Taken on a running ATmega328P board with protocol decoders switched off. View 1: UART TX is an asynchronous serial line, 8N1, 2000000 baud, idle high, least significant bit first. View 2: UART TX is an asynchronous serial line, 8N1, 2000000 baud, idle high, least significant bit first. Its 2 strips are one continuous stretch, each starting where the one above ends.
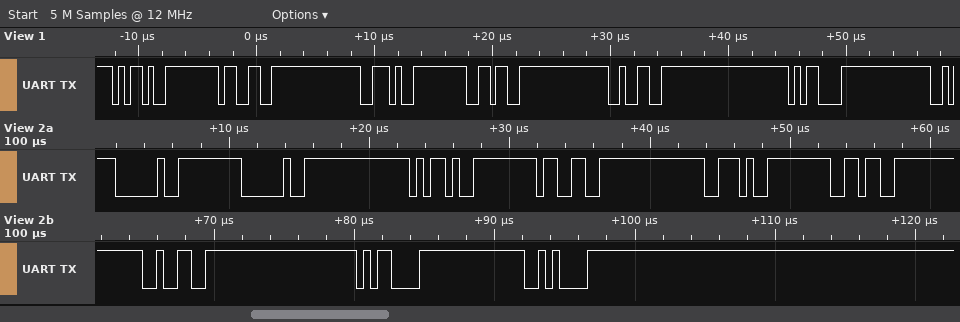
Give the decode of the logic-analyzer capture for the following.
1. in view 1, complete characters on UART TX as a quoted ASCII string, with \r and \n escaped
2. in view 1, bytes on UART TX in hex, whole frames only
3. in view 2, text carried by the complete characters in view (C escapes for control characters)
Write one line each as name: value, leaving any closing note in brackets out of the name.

in view 1, complete characters on UART TX as a quoted ASCII string, with \r and \n escaped: "-3.62\r"
in view 1, bytes on UART TX in hex, whole frames only: 0x2D 0x33 0x2E 0x36 0x32 0x0D
in view 2, text carried by the complete characters in view: "  -3.62\r\n"
